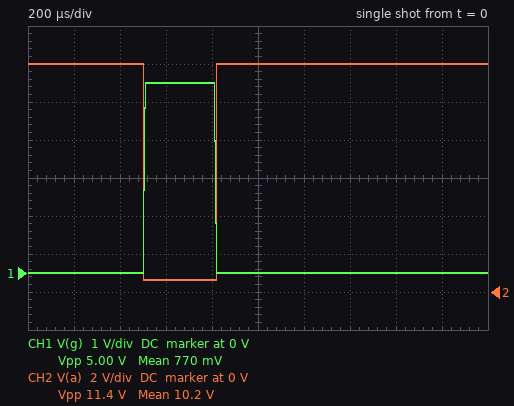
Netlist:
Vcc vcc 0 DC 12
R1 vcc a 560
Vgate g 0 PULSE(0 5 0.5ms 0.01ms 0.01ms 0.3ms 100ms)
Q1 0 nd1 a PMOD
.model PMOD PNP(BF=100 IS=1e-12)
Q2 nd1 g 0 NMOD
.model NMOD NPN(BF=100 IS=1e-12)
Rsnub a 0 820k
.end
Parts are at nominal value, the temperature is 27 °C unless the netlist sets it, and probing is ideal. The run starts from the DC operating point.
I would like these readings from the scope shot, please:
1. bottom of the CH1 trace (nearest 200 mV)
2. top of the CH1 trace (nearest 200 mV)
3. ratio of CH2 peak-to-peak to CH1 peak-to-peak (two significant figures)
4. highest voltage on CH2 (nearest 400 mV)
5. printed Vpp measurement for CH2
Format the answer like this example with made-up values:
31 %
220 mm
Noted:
0 V
5.0 V
2.3
12.0 V
11.4 V
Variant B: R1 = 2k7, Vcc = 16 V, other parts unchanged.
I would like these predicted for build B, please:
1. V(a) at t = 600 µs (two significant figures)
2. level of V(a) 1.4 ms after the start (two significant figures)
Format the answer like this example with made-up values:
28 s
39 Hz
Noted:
600 mV
16 V
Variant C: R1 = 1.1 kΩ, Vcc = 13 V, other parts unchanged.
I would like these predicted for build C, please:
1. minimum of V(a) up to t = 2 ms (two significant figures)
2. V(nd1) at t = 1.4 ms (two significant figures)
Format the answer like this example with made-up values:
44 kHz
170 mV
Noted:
620 mV
13 V
